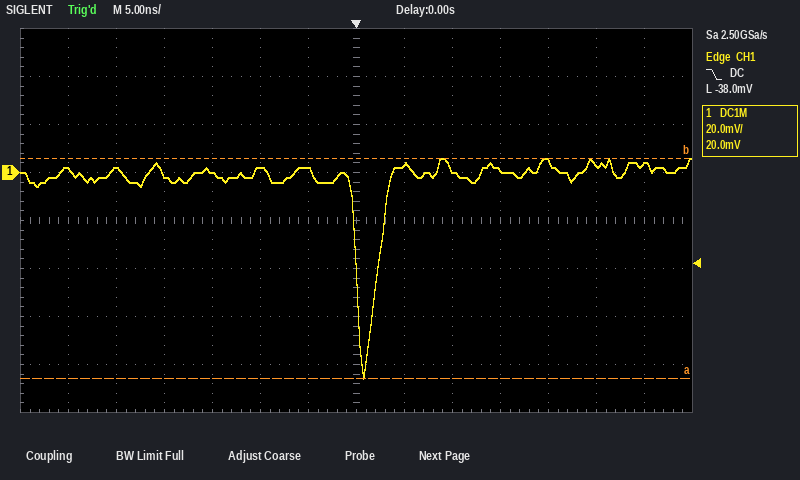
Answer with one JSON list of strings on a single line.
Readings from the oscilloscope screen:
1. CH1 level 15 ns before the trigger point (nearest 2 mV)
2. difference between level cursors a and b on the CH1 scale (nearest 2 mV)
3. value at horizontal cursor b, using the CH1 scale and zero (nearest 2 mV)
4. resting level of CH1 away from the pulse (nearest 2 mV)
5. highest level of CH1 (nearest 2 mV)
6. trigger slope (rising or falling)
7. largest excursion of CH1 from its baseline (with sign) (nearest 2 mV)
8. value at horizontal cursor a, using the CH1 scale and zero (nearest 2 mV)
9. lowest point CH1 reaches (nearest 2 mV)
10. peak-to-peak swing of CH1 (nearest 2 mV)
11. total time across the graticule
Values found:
["0 mV", "92 mV", "6 mV", "0 mV", "6 mV", "falling", "-86 mV", "-86 mV", "-86 mV", "92 mV", "70 ns"]
